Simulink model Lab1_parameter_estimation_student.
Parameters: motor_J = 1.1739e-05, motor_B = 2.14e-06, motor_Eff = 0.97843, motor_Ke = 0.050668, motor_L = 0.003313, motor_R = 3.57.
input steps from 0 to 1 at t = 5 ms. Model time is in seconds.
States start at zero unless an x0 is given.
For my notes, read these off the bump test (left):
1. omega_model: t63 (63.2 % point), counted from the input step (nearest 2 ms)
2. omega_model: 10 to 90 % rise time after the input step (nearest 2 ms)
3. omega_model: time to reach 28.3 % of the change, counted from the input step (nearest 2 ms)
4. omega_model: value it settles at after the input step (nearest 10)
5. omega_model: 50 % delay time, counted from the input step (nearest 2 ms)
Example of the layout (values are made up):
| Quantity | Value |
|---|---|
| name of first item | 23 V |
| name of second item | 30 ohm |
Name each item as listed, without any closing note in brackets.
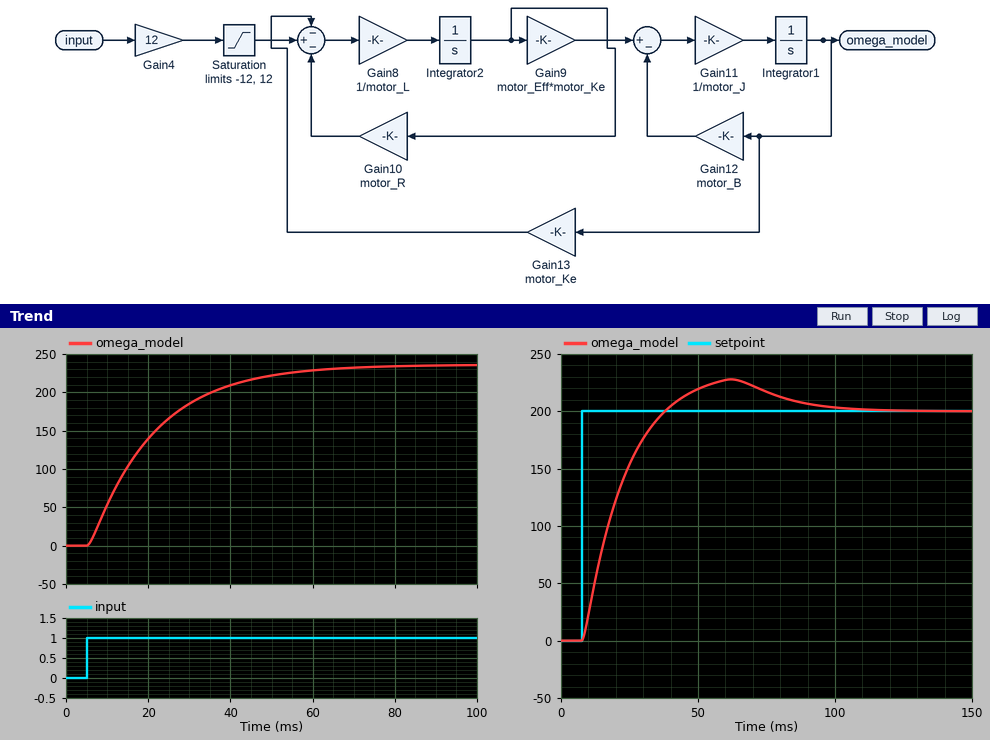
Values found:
| Quantity | Value |
|---|---|
| omega_model: t63 (63.2 % point), counted from the input step | 16 ms |
| omega_model: 10 to 90 % rise time after the input step | 34 ms |
| omega_model: time to reach 28.3 % of the change, counted from the input step | 6 ms |
| omega_model: value it settles at after the input step | 240 |
| omega_model: 50 % delay time, counted from the input step | 12 ms |
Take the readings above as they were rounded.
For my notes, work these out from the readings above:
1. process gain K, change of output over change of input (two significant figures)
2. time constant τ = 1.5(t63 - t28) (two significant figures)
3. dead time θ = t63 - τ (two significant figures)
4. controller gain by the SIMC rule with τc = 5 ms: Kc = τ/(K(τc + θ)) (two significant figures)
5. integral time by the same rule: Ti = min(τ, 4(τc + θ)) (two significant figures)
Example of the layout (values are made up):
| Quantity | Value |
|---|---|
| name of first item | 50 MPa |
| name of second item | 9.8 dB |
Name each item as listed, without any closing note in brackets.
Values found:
| Quantity | Value |
|---|---|
| process gain K, change of output over change of input | 240 |
| time constant τ = 1.5(t63 - t28) | 15 ms |
| dead time θ = t63 - τ | 1.0 ms |
| controller gain by the SIMC rule with τc = 5 ms: Kc = τ/(K(τc + θ)) | 0.010 |
| integral time by the same rule: Ti = min(τ, 4(τc + θ)) | 15 ms |
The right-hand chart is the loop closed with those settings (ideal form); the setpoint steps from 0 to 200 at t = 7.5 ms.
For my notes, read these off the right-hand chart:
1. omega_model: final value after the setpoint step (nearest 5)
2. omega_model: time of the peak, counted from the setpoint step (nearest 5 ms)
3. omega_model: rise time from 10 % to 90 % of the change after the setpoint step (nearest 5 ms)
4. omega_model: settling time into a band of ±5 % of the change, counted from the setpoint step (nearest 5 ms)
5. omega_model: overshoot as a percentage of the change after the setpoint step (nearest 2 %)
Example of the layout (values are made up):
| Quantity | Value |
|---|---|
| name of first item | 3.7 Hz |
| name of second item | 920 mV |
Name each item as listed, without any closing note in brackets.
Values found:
| Quantity | Value |
|---|---|
| omega_model: final value after the setpoint step | 200 |
| omega_model: time of the peak, counted from the setpoint step | 55 ms |
| omega_model: rise time from 10 % to 90 % of the change after the setpoint step | 20 ms |
| omega_model: settling time into a band of ±5 % of the change, counted from the setpoint step | 75 ms |
| omega_model: overshoot as a percentage of the change after the setpoint step | 14 % |
